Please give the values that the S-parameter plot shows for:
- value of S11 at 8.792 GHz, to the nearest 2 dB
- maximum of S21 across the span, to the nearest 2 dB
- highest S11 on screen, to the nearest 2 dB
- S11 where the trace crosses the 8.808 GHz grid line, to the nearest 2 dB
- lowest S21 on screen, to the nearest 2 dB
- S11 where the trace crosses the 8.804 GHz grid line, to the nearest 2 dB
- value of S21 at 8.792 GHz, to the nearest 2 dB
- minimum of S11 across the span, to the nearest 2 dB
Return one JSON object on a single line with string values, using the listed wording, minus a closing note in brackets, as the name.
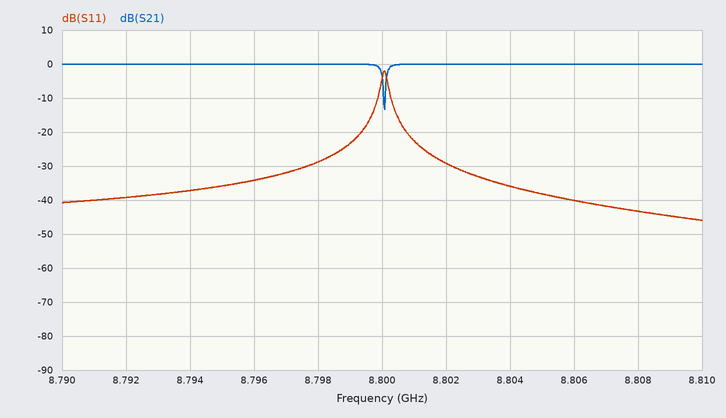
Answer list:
{"value of S11 at 8.792 GHz, to the nearest 2 dB": "-40 dB", "maximum of S21 across the span, to the nearest 2 dB": "0 dB", "highest S11 on screen, to the nearest 2 dB": "-2 dB", "S11 where the trace crosses the 8.808 GHz grid line, to the nearest 2 dB": "-44 dB", "lowest S21 on screen, to the nearest 2 dB": "-14 dB", "S11 where the trace crosses the 8.804 GHz grid line, to the nearest 2 dB": "-36 dB", "value of S21 at 8.792 GHz, to the nearest 2 dB": "0 dB", "minimum of S11 across the span, to the nearest 2 dB": "-46 dB"}
